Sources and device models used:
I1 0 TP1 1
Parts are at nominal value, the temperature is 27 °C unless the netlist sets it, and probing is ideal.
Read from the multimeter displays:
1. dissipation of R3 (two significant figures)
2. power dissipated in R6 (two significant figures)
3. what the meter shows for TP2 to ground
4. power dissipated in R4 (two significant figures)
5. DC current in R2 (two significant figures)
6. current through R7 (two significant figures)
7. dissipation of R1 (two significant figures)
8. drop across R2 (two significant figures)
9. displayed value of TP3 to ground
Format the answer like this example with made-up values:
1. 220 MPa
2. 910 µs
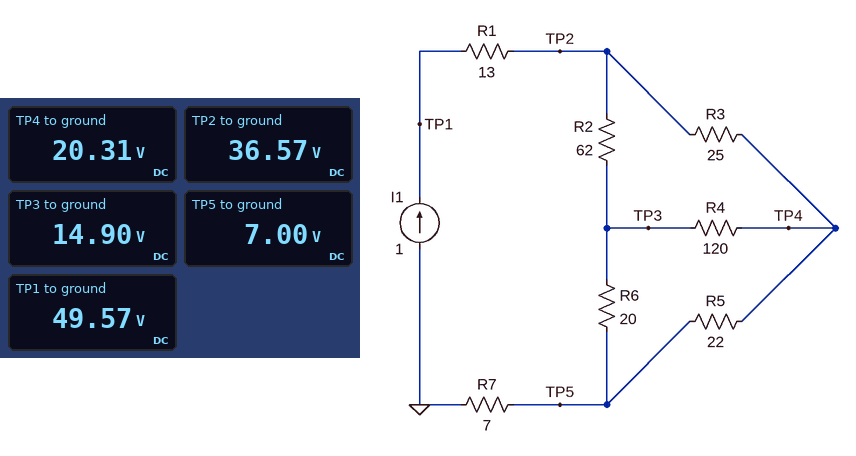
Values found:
1. 11 W
2. 3.1 W
3. 36.57 V
4. 240 mW
5. 350 mA
6. 1.0 A
7. 13 W
8. 22 V
9. 14.90 V
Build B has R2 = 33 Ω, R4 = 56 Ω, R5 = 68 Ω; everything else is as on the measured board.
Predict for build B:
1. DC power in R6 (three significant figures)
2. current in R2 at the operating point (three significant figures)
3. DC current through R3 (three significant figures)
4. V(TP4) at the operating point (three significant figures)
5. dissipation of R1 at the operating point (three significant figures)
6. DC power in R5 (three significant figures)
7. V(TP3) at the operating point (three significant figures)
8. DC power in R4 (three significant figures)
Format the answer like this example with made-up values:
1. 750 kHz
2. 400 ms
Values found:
1. 9.50 W
2. 558 mA
3. 442 mA
4. 28.1 V
5. 13.0 W
6. 6.57 W
7. 20.8 V
8. 966 mW
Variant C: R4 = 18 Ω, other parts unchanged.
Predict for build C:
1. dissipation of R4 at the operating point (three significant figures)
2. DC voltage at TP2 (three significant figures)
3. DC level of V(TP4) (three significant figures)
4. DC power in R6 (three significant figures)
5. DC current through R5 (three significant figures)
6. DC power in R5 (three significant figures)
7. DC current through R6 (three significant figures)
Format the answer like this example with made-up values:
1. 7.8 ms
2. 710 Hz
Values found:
1. 376 mW
2. 35.9 V
3. 18.8 V
4. 4.27 W
5. 538 mA
6. 6.37 W
7. 462 mA
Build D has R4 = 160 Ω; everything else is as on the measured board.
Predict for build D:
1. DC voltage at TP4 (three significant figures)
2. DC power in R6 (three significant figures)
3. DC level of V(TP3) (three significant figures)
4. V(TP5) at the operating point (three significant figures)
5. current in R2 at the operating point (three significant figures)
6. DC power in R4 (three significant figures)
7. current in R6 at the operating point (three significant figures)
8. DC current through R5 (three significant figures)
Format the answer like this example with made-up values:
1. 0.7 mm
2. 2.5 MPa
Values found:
1. 20.5 V
2. 3.02 W
3. 14.8 V
4. 7.00 V
5. 353 mA
6. 202 mW
7. 388 mA
8. 612 mA
